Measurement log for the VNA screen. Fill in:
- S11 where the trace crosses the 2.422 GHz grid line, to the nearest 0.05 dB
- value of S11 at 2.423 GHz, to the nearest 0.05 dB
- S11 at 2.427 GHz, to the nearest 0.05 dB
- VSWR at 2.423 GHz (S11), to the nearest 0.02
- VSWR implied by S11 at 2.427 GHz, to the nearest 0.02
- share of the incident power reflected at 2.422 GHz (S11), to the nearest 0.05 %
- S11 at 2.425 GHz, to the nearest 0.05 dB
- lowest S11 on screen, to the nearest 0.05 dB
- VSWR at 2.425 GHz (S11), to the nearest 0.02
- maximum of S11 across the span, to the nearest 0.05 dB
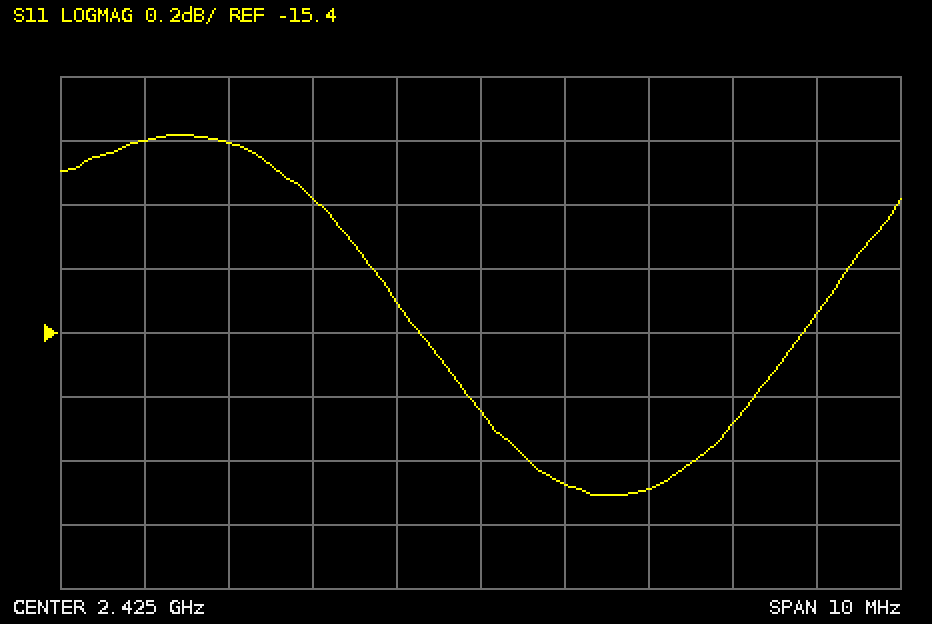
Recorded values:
-14.80 dB
-15.00 dB
-15.90 dB
1.44
1.38
3.30 %
-15.65 dB
-15.90 dB
1.40
-14.80 dB
